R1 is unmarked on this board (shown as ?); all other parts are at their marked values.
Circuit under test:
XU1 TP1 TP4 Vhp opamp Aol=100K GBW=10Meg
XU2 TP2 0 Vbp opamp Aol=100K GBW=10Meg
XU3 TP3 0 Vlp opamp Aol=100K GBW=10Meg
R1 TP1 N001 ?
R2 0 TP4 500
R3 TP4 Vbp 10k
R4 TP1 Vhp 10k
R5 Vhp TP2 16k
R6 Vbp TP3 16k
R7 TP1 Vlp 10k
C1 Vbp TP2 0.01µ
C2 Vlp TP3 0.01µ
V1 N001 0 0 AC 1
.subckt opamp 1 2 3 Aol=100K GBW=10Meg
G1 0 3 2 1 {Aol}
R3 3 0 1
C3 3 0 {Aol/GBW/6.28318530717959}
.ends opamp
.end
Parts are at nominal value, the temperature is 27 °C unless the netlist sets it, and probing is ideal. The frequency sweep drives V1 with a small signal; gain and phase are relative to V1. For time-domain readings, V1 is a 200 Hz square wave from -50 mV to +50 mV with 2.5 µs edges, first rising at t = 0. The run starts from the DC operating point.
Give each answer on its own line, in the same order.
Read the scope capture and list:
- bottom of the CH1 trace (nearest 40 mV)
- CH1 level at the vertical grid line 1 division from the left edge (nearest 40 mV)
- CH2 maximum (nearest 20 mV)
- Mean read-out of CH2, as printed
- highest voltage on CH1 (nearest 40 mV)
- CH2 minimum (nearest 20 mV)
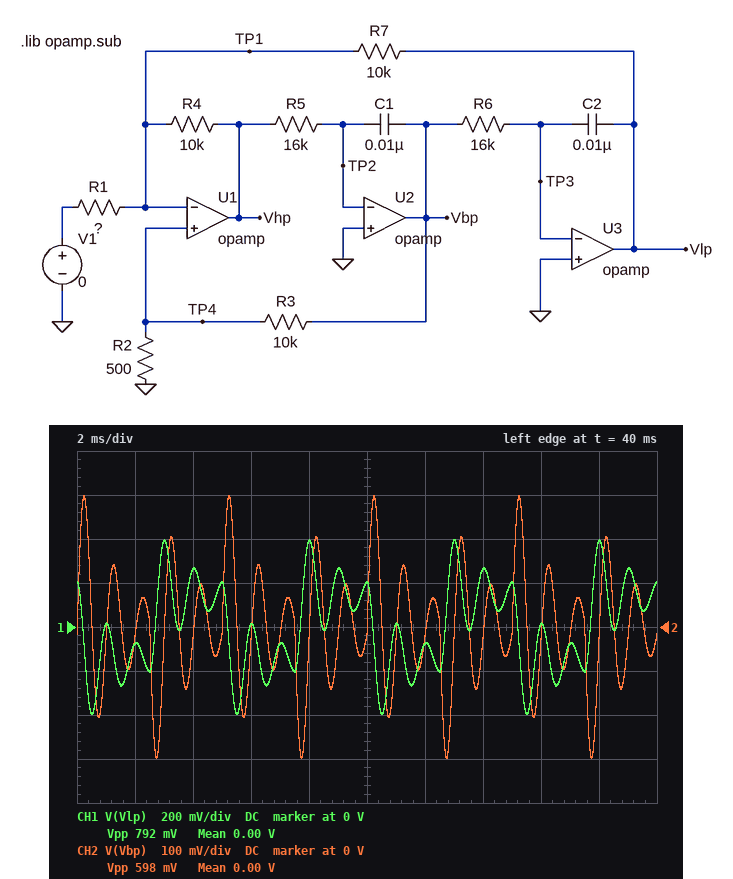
-400 mV
-80 mV
300 mV
0.00 V
400 mV
-300 mV
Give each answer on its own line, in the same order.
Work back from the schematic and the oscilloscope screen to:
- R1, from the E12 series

3.3 kΩ
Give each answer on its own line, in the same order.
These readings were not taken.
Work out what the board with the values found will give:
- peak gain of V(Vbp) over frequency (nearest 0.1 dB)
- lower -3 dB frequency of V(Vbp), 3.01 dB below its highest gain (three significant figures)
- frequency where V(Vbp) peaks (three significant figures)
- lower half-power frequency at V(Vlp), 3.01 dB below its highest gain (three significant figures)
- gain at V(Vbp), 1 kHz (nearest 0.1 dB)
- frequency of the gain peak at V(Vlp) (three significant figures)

22.1 dB
883 Hz
995 Hz
852 Hz
22.1 dB
980 Hz
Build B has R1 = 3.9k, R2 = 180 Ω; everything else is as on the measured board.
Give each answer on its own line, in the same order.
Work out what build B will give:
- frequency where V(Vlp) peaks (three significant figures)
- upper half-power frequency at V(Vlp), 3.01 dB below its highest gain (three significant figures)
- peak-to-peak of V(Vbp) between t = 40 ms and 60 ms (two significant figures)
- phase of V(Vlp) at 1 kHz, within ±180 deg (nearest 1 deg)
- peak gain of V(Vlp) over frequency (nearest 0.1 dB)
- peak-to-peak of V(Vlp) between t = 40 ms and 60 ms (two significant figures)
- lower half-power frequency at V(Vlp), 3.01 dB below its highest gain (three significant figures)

993 Hz
1.03 kHz
1.0 V
82 deg
30.1 dB
1.2 V
952 Hz
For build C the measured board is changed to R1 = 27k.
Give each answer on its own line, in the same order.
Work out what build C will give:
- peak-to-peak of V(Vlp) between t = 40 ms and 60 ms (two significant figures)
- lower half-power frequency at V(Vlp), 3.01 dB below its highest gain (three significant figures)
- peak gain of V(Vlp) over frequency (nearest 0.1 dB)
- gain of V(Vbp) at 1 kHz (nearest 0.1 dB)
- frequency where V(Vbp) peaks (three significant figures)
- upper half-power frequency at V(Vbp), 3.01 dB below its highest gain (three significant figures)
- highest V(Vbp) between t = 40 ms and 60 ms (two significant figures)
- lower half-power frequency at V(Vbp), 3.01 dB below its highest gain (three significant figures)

140 mV
934 Hz
10.4 dB
10.3 dB
995 Hz
1.05 kHz
57 mV
940 Hz
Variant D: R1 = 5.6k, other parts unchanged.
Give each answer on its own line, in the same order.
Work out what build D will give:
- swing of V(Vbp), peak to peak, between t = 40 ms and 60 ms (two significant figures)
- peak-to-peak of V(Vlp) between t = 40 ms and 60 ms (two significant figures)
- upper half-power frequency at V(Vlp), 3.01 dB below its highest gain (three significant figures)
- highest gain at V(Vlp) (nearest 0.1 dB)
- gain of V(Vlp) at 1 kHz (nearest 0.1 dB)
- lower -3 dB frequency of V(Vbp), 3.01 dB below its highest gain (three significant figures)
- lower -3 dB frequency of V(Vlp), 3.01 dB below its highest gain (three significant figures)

410 mV
530 mV
1.07 kHz
20.0 dB
19.9 dB
909 Hz
892 Hz
